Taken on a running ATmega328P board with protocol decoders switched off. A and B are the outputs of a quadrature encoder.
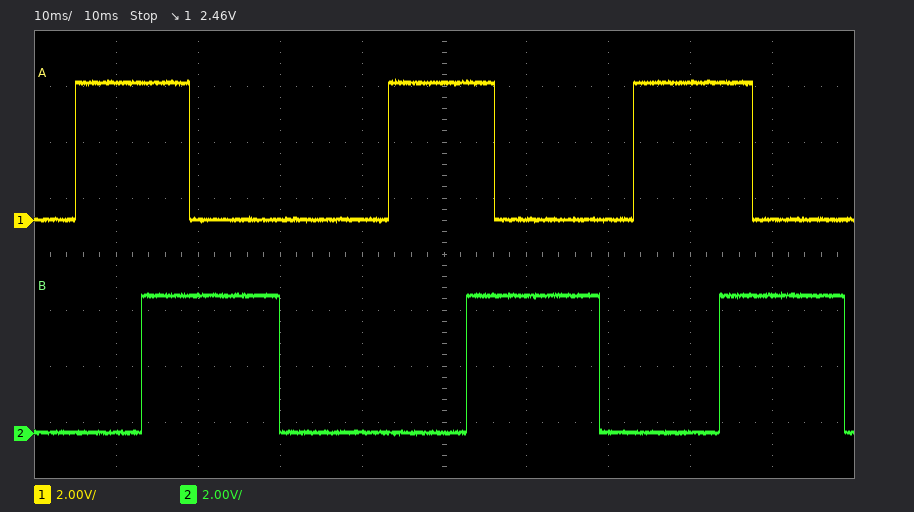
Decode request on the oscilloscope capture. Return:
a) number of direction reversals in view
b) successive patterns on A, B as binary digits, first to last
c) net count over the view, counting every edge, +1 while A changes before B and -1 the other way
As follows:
0
00 10 11 01 00 10 11 01 00 10 11 01 00
+12
